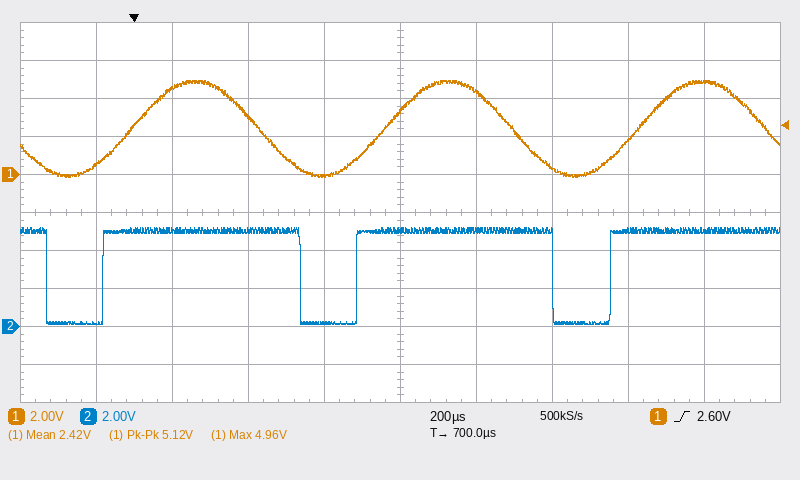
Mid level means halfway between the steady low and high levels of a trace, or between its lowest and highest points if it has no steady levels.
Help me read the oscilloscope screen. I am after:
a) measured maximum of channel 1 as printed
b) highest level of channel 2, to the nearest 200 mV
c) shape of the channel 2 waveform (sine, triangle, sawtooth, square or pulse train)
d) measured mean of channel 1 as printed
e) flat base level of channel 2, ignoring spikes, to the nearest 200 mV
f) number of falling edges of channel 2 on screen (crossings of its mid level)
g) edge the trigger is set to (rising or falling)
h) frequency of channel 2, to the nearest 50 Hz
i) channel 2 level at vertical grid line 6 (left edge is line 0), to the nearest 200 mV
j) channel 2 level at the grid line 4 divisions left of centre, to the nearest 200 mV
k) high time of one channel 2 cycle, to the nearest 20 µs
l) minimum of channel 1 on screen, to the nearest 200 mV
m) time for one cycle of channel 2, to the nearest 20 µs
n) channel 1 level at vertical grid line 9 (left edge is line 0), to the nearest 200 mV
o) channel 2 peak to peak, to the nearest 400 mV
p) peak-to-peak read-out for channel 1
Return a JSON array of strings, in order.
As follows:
["4.96 V", "5.2 V", "pulse train", "2.42 V", "200 mV", "3", "rising", "1.50 kHz", "5.0 V", "200 mV", "520 µs", "-200 mV", "660 µs", "4.8 V", "5.2 V", "5.12 V"]
